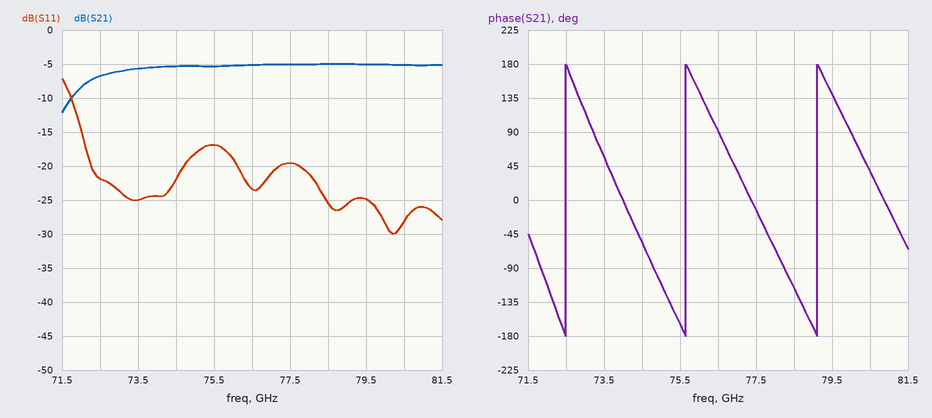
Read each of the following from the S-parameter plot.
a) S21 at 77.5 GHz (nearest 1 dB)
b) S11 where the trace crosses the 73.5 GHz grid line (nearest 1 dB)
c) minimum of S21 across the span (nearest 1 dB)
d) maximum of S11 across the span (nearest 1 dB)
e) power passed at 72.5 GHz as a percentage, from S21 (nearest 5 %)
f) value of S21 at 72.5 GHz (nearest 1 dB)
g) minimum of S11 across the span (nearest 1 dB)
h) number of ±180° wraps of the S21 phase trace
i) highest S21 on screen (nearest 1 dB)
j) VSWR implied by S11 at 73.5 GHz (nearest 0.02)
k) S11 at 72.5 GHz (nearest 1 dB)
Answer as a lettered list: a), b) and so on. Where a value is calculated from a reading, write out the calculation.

a) -5 dB
b) -25 dB
c) -12 dB
d) -7 dB
e) 10^(-7/10) ≈ 20 %
f) -7 dB
g) -30 dB
h) 3
i) -5 dB
j) |Γ| = 10^(-25/20) = 0.0562; VSWR = (1 + 0.0562)/(1 − 0.0562) ≈ 1.12
k) -22 dB
